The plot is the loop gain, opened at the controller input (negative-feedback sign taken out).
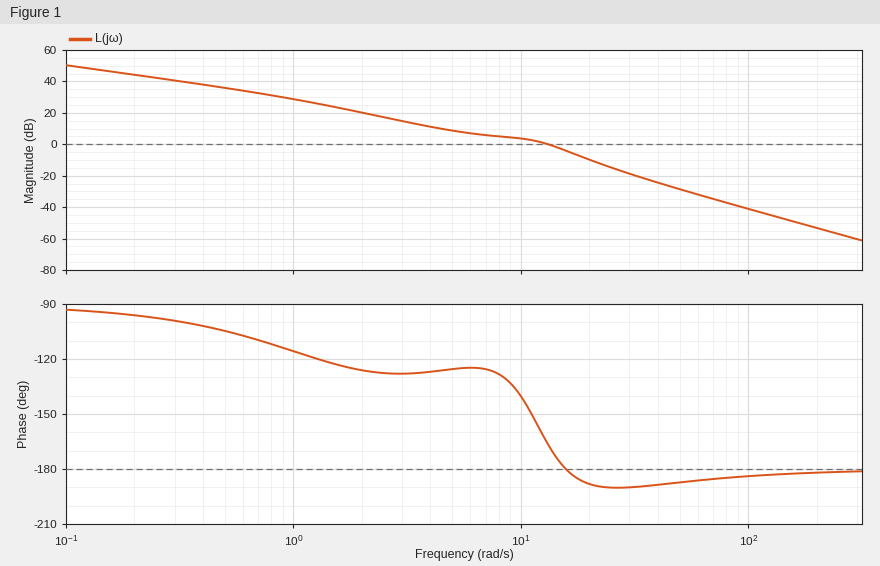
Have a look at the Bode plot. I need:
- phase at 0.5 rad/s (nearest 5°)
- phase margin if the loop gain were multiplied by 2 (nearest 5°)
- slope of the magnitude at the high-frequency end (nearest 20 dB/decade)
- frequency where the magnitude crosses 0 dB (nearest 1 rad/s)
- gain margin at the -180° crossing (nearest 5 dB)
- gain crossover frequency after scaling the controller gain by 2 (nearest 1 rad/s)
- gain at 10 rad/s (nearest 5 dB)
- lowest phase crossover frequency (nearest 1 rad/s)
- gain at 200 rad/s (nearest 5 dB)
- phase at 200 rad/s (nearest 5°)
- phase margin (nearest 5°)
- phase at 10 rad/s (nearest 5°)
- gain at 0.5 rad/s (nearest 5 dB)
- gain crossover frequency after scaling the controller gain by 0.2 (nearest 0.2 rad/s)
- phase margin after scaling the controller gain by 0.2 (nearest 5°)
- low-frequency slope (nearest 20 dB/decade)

-105°
-5°
-40 dB/decade
13 rad/s
5 dB
17 rad/s
5 dB
16 rad/s
-55 dB
-180°
15°
-140°
35 dB
3.2 rad/s
50°
-20 dB/decade
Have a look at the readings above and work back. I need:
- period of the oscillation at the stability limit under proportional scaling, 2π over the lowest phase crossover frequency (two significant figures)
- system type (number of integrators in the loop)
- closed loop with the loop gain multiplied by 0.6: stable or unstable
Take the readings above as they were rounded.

0.39 s
1
stable
